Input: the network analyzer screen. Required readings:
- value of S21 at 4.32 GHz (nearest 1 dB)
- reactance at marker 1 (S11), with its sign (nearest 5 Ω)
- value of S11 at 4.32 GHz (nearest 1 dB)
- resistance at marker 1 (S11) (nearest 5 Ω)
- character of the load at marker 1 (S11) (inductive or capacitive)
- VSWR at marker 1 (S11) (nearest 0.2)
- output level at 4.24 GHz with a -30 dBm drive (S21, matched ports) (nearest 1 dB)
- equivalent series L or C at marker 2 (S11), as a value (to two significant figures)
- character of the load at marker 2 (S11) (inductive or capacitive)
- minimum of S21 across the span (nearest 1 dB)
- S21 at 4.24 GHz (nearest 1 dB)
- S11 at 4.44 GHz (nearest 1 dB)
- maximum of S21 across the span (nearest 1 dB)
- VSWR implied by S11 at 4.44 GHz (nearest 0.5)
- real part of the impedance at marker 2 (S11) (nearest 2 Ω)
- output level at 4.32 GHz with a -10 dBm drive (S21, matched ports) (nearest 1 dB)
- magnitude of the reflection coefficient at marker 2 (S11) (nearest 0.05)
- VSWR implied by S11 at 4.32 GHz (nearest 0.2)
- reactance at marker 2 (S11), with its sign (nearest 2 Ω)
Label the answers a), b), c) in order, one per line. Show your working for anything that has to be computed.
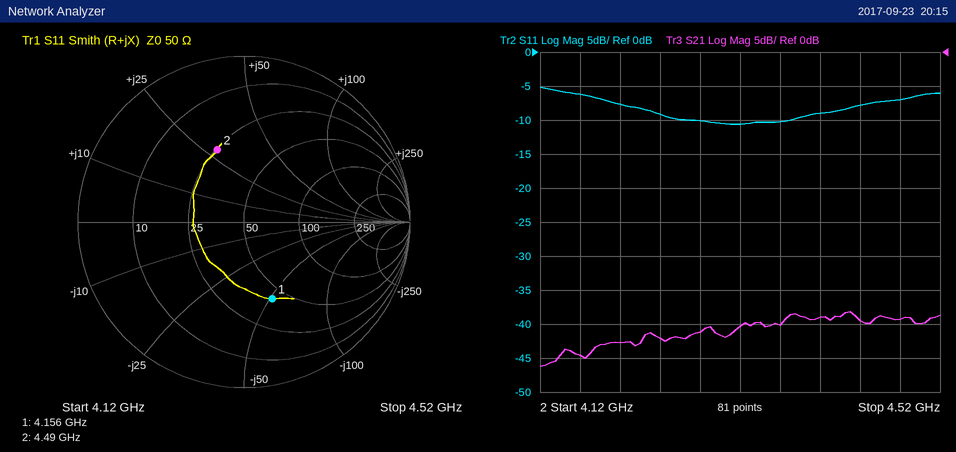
a) -40 dB
b) -50 Ω
c) -11 dB
d) 40 Ω
e) capacitive
f) 3.0
g) -30 dBm + (-42 dB) = -72 dBm
h) L = 28 Ω/(2π × 4.49 GHz) ≈ 1.0 nH
i) inductive
j) -46 dB
k) -42 dB
l) -8 dB
m) -38 dB
n) |Γ| = 10^(-8/20) = 0.3981; VSWR = (1 + 0.3981)/(1 − 0.3981) ≈ 2.32, so 2.5 to the nearest 0.5
o) 26 Ω
p) -10 dBm + (-40 dB) = -50 dBm
q) 0.45
r) |Γ| = 10^(-11/20) = 0.2818; VSWR = (1 + 0.2818)/(1 − 0.2818) ≈ 1.8
s) +28 Ω
